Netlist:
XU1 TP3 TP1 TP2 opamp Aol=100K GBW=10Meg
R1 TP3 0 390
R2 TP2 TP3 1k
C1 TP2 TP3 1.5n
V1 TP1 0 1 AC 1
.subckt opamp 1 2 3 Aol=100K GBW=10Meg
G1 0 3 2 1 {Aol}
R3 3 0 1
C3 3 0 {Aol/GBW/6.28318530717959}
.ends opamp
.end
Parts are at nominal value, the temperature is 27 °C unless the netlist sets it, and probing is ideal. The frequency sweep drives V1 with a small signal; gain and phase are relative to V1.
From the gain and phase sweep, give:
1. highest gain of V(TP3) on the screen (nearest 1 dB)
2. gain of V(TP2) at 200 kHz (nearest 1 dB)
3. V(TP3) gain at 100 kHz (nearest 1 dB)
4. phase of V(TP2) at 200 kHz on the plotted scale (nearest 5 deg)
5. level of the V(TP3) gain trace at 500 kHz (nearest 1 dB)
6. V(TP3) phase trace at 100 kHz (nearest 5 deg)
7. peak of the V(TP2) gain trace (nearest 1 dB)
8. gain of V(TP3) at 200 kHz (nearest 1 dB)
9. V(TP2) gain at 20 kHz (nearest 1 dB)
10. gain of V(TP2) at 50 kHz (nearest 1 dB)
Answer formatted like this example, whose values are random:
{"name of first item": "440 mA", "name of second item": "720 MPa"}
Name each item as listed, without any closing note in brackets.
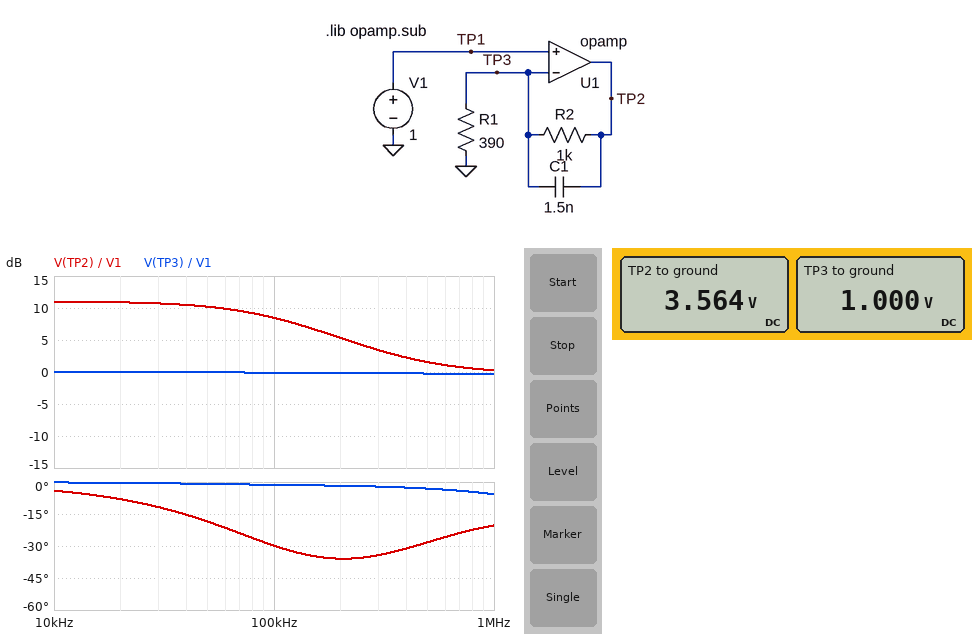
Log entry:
{"highest gain of V(TP3) on the screen": "0 dB", "gain of V(TP2) at 200 kHz": "5 dB", "V(TP3) gain at 100 kHz": "0 dB", "phase of V(TP2) at 200 kHz on the plotted scale": "-35 deg", "level of the V(TP3) gain trace at 500 kHz": "0 dB", "V(TP3) phase trace at 100 kHz": "0 deg", "peak of the V(TP2) gain trace": "11 dB", "gain of V(TP3) at 200 kHz": "0 dB", "V(TP2) gain at 20 kHz": "11 dB", "gain of V(TP2) at 50 kHz": "10 dB"}
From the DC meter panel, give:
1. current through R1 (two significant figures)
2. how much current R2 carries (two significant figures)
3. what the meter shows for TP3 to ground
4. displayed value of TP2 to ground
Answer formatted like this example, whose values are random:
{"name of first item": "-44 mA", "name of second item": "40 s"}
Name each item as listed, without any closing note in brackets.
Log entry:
{"current through R1": "2.6 mA", "how much current R2 carries": "2.6 mA", "what the meter shows for TP3 to ground": "1.000 V", "displayed value of TP2 to ground": "3.564 V"}
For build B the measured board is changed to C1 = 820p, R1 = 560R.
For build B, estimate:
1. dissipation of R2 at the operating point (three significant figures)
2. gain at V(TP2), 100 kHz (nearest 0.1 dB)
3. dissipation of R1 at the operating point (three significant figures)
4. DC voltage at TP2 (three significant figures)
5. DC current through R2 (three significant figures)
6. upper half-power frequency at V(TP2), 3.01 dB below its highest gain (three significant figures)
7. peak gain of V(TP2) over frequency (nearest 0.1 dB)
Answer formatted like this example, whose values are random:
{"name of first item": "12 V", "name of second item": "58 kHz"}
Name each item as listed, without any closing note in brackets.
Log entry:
{"dissipation of R2 at the operating point": "3.19 mW", "gain at V(TP2), 100 kHz": "8.0 dB", "dissipation of R1 at the operating point": "1.79 mW", "DC voltage at TP2": "2.79 V", "DC current through R2": "1.79 mA", "upper half-power frequency at V(TP2), 3.01 dB below its highest gain": "215 kHz", "peak gain of V(TP2) over frequency": "8.9 dB"}
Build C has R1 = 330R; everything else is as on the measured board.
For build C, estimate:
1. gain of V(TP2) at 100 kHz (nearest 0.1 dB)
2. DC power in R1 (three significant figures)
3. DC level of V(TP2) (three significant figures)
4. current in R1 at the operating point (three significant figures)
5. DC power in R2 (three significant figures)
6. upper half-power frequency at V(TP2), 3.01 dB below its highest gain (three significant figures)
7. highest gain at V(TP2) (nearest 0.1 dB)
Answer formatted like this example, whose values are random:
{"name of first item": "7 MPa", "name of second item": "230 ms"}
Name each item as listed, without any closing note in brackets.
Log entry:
{"gain of V(TP2) at 100 kHz": "9.4 dB", "DC power in R1": "3.03 mW", "DC level of V(TP2)": "4.03 V", "current in R1 at the operating point": "3.03 mA", "DC power in R2": "9.18 mW", "upper half-power frequency at V(TP2), 3.01 dB below its highest gain": "109 kHz", "highest gain at V(TP2)": "12.1 dB"}
